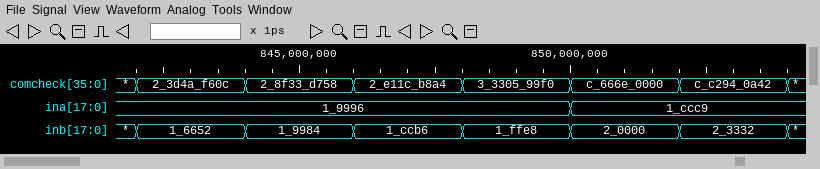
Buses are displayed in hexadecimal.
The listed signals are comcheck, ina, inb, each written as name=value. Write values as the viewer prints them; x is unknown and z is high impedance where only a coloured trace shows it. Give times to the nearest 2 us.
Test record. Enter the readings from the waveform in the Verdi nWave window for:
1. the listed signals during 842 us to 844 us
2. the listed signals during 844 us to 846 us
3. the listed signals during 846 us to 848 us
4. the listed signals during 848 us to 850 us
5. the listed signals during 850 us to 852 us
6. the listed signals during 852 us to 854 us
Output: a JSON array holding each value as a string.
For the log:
["comcheck=2_3d4a_f60c, ina=1_9996, inb=1_6652", "comcheck=2_8f33_d758, ina=1_9996, inb=1_9984", "comcheck=2_e11c_b8a4, ina=1_9996, inb=1_ccb6", "comcheck=3_3305_99f0, ina=1_9996, inb=1_ffe8", "comcheck=c_666e_0000, ina=1_ccc9, inb=2_0000", "comcheck=c_c294_0a42, ina=1_ccc9, inb=2_3332"]
